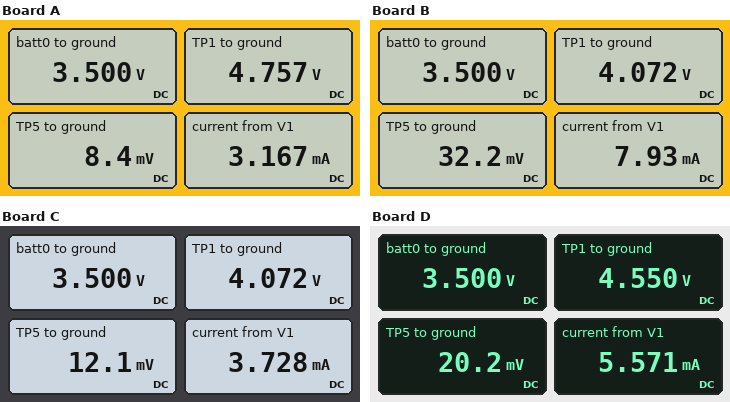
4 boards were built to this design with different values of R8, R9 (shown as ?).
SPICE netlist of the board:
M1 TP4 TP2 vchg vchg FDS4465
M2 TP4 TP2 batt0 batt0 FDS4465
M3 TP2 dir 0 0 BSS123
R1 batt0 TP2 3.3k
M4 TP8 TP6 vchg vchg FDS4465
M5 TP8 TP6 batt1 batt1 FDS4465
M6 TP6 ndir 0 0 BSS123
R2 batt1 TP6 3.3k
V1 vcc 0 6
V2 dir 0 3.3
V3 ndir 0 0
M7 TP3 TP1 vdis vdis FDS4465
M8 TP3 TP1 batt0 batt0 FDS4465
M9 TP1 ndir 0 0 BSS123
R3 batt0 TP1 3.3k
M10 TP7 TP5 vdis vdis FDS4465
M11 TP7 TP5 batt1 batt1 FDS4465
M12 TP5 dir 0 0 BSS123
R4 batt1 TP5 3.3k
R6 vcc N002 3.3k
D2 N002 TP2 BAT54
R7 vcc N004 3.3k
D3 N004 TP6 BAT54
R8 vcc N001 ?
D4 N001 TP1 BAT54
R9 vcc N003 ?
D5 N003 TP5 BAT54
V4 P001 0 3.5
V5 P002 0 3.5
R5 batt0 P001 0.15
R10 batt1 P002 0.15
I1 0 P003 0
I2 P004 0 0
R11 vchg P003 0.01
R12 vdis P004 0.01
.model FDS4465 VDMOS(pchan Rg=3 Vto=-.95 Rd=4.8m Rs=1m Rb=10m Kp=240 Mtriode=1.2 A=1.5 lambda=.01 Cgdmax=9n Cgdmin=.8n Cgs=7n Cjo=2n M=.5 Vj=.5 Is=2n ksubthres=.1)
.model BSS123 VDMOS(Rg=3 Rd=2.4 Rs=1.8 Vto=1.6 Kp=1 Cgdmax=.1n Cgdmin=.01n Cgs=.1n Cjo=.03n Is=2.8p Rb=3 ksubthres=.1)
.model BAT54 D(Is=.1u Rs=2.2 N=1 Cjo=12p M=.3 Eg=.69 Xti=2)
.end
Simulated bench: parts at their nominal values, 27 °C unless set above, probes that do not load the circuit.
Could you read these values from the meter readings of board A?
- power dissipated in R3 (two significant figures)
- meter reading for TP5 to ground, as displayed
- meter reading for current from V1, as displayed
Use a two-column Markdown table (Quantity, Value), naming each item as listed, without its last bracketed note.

| Quantity | Value |
|---|---|
| power dissipated in R3 | 480 µW |
| meter reading for TP5 to ground, as displayed | 8.4 mV |
| meter reading for current from V1, as displayed | 3.167 mA |
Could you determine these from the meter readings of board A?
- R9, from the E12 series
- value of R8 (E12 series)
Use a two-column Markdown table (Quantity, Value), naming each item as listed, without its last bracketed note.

| Quantity | Value |
|---|---|
| R9, from the E12 series | 8.2 kΩ |
| value of R8 | 2.7 kΩ |
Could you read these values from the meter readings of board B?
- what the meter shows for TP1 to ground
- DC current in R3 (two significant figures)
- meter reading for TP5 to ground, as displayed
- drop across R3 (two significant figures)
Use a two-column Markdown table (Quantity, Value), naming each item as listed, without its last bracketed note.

| Quantity | Value |
|---|---|
| what the meter shows for TP1 to ground | 4.072 V |
| DC current in R3 | 170 µA |
| meter reading for TP5 to ground, as displayed | 32.2 mV |
| drop across R3 | 570 mV |
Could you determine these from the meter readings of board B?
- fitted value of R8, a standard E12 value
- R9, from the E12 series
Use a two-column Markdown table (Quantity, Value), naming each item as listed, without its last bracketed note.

| Quantity | Value |
|---|---|
| fitted value of R8, a standard E12 value | 10 kΩ |
| R9, from the E12 series | 1 kΩ |
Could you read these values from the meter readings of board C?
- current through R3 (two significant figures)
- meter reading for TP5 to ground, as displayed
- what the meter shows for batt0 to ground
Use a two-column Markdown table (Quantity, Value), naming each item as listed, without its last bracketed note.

| Quantity | Value |
|---|---|
| current through R3 | 170 µA |
| meter reading for TP5 to ground, as displayed | 12.1 mV |
| what the meter shows for batt0 to ground | 3.500 V |
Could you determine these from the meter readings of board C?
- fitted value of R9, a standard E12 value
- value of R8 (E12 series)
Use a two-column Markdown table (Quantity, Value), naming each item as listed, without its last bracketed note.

| Quantity | Value |
|---|---|
| fitted value of R9, a standard E12 value | 3.9 kΩ |
| value of R8 | 10 kΩ |
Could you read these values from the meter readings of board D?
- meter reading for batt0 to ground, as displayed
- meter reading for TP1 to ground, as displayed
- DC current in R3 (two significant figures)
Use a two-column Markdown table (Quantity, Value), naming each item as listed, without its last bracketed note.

| Quantity | Value |
|---|---|
| meter reading for batt0 to ground, as displayed | 3.500 V |
| meter reading for TP1 to ground, as displayed | 4.550 V |
| DC current in R3 | 320 µA |
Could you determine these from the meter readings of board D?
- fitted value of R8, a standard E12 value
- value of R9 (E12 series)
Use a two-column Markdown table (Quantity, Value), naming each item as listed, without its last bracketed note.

| Quantity | Value |
|---|---|
| fitted value of R8, a standard E12 value | 3.9 kΩ |
| value of R9 | 1.8 kΩ |
